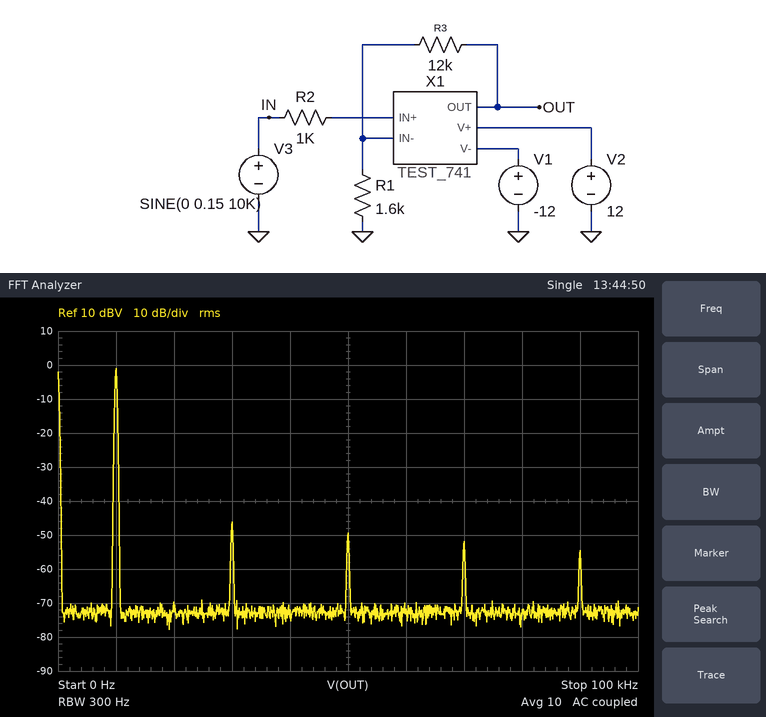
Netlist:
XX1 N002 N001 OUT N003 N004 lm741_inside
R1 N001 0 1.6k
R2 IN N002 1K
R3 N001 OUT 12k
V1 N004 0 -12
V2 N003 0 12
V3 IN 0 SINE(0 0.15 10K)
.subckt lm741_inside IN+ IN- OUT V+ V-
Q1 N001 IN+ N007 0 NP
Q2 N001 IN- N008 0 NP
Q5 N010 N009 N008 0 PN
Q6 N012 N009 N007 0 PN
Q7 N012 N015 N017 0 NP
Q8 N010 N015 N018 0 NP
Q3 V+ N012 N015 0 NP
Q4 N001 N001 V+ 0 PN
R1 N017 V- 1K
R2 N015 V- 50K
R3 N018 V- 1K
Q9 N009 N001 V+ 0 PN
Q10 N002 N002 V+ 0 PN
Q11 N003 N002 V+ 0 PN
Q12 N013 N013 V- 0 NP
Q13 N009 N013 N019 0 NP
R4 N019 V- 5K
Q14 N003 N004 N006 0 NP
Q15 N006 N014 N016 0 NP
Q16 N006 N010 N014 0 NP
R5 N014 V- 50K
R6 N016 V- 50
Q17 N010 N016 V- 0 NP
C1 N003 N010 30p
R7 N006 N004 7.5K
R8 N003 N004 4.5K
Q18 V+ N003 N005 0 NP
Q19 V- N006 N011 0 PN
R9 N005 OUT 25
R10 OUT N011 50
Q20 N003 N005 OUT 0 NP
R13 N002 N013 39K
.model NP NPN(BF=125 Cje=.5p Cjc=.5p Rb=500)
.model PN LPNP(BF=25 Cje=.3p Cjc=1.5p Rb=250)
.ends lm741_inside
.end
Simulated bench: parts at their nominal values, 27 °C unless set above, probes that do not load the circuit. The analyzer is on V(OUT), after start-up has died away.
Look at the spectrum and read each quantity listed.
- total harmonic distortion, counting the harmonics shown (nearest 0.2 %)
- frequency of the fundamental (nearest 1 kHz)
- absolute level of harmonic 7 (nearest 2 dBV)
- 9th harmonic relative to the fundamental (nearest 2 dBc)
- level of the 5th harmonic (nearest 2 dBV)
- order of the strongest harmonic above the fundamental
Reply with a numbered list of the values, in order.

1. 0.8 %
2. 10 kHz
3. -52 dBV
4. -54 dBc
5. -50 dBV
6. 3
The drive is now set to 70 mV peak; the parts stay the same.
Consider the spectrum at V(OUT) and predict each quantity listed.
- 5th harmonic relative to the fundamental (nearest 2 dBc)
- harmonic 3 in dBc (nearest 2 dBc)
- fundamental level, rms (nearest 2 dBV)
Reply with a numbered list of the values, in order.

1. -46 dBc
2. -42 dBc
3. -8 dBV
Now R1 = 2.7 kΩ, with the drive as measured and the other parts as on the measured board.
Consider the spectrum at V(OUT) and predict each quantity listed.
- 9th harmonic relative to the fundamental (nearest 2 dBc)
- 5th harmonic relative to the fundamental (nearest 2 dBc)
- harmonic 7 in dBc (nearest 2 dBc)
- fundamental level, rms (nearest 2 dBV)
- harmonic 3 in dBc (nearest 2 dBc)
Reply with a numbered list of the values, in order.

1. -56 dBc
2. -50 dBc
3. -54 dBc
4. -4 dBV
5. -48 dBc
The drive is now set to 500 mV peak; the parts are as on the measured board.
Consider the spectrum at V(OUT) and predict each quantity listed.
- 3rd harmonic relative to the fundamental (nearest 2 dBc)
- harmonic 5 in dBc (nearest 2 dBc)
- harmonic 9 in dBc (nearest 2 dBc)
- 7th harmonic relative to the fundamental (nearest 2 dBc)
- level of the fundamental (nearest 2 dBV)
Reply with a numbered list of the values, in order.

1. -46 dBc
2. -52 dBc
3. -56 dBc
4. -54 dBc
5. 10 dBV
